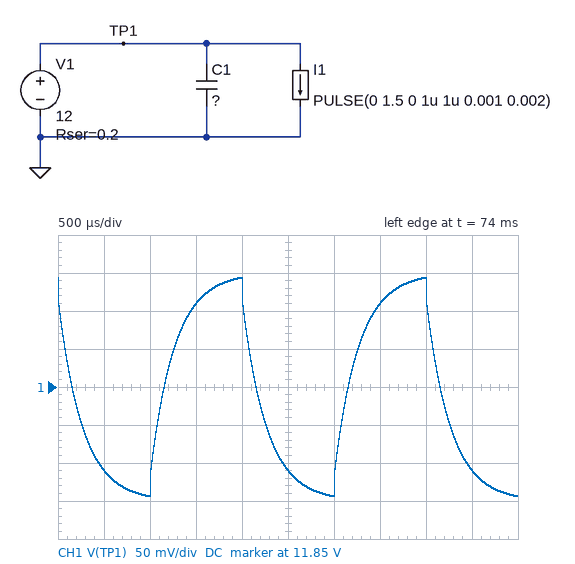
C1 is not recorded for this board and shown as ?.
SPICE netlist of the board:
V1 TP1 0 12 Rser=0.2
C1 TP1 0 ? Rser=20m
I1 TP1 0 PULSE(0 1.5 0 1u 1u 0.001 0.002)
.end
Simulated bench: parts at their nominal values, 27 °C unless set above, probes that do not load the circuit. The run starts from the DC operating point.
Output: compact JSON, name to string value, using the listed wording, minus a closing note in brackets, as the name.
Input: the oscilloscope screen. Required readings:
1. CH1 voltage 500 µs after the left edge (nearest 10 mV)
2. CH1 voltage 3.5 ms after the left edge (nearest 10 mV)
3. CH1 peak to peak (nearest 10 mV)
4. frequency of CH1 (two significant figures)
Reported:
{"CH1 voltage 500 µs after the left edge": "11.74 V", "CH1 voltage 3.5 ms after the left edge": "11.96 V", "CH1 peak to peak": "290 mV", "frequency of CH1": "500 Hz"}
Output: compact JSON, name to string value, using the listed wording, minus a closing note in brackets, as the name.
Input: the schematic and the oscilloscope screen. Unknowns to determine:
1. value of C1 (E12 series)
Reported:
{"value of C1": "1.2 mF"}
